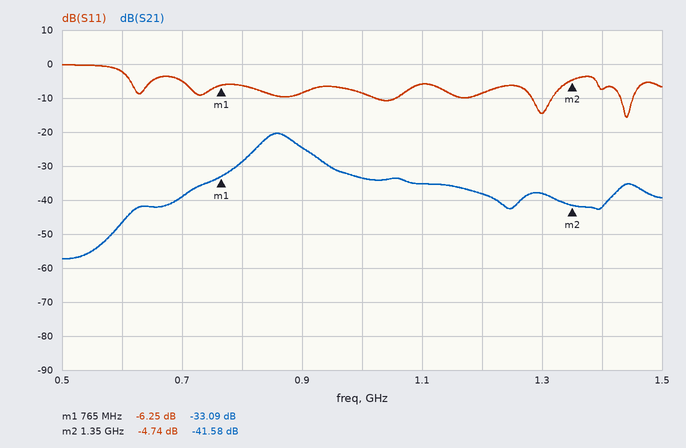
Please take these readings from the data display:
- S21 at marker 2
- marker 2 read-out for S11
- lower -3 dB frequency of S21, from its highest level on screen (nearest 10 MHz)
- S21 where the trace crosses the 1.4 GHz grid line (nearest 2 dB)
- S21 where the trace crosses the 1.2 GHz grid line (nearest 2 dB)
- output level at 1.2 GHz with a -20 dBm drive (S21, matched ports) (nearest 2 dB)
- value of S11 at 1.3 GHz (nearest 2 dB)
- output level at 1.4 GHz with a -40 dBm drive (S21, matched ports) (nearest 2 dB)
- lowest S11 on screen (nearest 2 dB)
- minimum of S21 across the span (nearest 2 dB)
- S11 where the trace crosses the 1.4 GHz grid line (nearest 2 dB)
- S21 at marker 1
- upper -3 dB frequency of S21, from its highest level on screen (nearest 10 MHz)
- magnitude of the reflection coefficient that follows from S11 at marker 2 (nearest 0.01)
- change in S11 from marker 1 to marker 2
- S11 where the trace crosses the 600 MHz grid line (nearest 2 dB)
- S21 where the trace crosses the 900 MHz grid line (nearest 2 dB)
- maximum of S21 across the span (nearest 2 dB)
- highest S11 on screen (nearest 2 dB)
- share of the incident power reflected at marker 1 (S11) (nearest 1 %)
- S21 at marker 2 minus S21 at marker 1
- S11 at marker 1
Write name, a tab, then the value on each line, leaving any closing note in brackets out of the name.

S21 at marker 2	-41.58 dB
marker 2 read-out for S11	-4.74 dB
lower -3 dB frequency of S21, from its highest level on screen	830 MHz
S21 where the trace crosses the 1.4 GHz grid line	-42 dB
S21 where the trace crosses the 1.2 GHz grid line	-38 dB
output level at 1.2 GHz with a -20 dBm drive (S21, matched ports)	-58 dBm
value of S11 at 1.3 GHz	-14 dB
output level at 1.4 GHz with a -40 dBm drive (S21, matched ports)	-82 dBm
lowest S11 on screen	-16 dB
minimum of S21 across the span	-58 dB
S11 where the trace crosses the 1.4 GHz grid line	-8 dB
S21 at marker 1	-33.09 dB
upper -3 dB frequency of S21, from its highest level on screen	890 MHz
magnitude of the reflection coefficient that follows from S11 at marker 2	0.58
change in S11 from marker 1 to marker 2	1.51 dB
S11 where the trace crosses the 600 MHz grid line	-2 dB
S21 where the trace crosses the 900 MHz grid line	-24 dB
maximum of S21 across the span	-20 dB
highest S11 on screen	0 dB
share of the incident power reflected at marker 1 (S11)	24 %
S21 at marker 2 minus S21 at marker 1	-8.49 dB
S11 at marker 1	-6.25 dB
